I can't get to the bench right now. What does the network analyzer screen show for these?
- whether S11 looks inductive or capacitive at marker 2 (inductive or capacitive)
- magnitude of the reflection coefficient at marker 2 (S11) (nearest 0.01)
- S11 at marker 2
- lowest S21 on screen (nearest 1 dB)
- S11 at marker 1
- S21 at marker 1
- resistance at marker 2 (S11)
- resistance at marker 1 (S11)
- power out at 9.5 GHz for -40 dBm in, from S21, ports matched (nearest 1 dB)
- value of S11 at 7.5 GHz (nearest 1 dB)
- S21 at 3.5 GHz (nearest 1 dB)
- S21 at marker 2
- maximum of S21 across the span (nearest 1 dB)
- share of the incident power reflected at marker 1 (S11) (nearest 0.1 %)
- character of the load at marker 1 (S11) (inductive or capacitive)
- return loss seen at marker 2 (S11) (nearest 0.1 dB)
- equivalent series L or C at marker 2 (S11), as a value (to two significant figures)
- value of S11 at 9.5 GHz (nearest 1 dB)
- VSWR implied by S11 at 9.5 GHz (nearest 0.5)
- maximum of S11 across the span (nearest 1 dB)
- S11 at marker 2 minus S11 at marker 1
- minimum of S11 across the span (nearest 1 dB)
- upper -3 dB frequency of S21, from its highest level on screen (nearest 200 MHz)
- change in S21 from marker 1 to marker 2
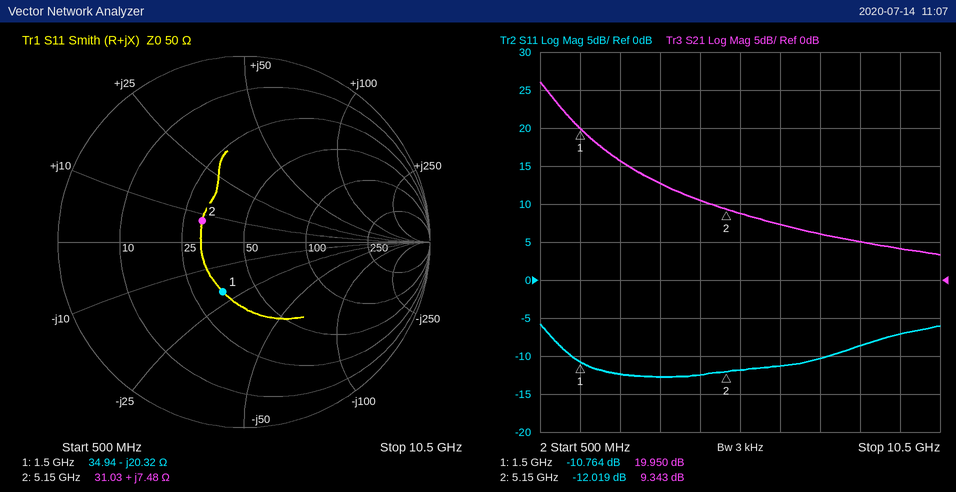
inductive
0.25
-12.019 dB
3 dB
-10.764 dB
19.950 dB
31.03 Ω
34.94 Ω
-36 dBm
-10 dB
13 dB
9.343 dB
26 dB
8.4 %
capacitive
12.0 dB
230 pH
-7 dB
2.5
-6 dB
-1.255 dB
-13 dB
1.0 GHz
-10.607 dB
